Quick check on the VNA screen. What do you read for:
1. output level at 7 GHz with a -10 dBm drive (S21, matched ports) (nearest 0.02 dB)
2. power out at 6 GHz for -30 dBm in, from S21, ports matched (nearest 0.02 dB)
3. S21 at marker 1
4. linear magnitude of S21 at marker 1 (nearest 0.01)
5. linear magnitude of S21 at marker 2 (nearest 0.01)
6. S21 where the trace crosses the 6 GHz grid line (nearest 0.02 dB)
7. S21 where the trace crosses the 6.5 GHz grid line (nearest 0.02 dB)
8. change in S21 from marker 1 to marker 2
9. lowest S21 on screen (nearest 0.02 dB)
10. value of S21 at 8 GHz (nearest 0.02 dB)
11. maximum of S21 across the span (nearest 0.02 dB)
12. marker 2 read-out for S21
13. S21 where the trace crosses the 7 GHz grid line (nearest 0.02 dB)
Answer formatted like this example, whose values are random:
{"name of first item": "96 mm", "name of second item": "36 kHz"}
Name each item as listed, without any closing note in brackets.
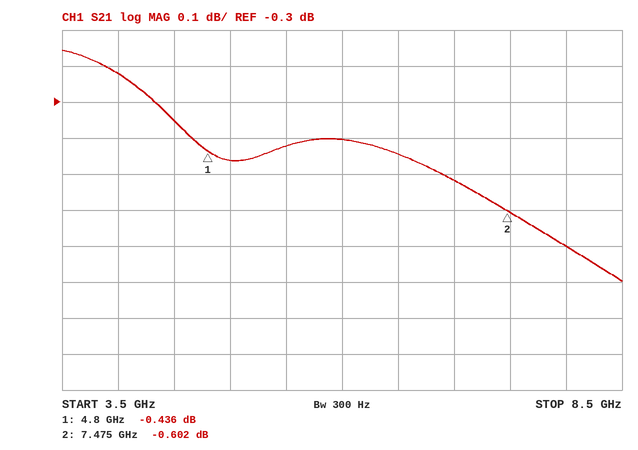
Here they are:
{"output level at 7 GHz with a -10 dBm drive (S21, matched ports)": "-10.52 dBm", "power out at 6 GHz for -30 dBm in, from S21, ports matched": "-30.40 dBm", "S21 at marker 1": "-0.436 dB", "linear magnitude of S21 at marker 1": "0.95", "linear magnitude of S21 at marker 2": "0.93", "S21 where the trace crosses the 6 GHz grid line": "-0.40 dB", "S21 where the trace crosses the 6.5 GHz grid line": "-0.44 dB", "change in S21 from marker 1 to marker 2": "-0.166 dB", "lowest S21 on screen": "-0.80 dB", "value of S21 at 8 GHz": "-0.70 dB", "maximum of S21 across the span": "-0.16 dB", "marker 2 read-out for S21": "-0.602 dB", "S21 where the trace crosses the 7 GHz grid line": "-0.52 dB"}
